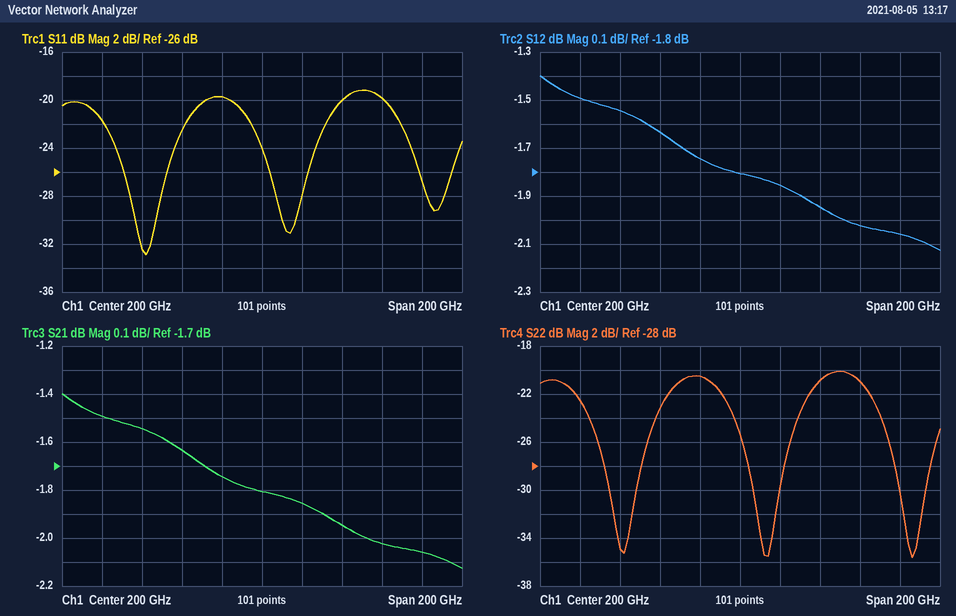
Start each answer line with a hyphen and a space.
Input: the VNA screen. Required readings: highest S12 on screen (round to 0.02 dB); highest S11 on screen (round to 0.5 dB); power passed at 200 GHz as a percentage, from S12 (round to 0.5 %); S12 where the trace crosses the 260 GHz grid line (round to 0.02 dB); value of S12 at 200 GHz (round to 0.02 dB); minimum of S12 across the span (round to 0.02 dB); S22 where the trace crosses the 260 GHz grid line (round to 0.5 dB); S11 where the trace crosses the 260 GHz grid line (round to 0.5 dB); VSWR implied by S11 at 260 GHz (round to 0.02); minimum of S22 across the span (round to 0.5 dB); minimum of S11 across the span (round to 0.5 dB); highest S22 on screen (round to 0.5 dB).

- -1.40 dB
- -19.0 dB
- 66.0 %
- -2.02 dB
- -1.80 dB
- -2.12 dB
- -21.0 dB
- -20.0 dB
- 1.22
- -35.5 dB
- -33.0 dB
- -20.0 dB
